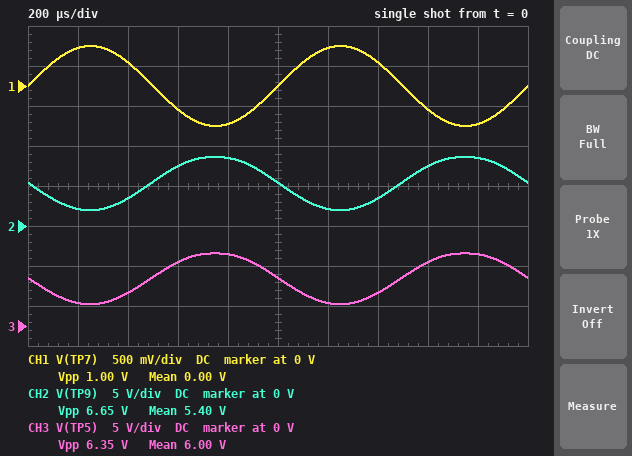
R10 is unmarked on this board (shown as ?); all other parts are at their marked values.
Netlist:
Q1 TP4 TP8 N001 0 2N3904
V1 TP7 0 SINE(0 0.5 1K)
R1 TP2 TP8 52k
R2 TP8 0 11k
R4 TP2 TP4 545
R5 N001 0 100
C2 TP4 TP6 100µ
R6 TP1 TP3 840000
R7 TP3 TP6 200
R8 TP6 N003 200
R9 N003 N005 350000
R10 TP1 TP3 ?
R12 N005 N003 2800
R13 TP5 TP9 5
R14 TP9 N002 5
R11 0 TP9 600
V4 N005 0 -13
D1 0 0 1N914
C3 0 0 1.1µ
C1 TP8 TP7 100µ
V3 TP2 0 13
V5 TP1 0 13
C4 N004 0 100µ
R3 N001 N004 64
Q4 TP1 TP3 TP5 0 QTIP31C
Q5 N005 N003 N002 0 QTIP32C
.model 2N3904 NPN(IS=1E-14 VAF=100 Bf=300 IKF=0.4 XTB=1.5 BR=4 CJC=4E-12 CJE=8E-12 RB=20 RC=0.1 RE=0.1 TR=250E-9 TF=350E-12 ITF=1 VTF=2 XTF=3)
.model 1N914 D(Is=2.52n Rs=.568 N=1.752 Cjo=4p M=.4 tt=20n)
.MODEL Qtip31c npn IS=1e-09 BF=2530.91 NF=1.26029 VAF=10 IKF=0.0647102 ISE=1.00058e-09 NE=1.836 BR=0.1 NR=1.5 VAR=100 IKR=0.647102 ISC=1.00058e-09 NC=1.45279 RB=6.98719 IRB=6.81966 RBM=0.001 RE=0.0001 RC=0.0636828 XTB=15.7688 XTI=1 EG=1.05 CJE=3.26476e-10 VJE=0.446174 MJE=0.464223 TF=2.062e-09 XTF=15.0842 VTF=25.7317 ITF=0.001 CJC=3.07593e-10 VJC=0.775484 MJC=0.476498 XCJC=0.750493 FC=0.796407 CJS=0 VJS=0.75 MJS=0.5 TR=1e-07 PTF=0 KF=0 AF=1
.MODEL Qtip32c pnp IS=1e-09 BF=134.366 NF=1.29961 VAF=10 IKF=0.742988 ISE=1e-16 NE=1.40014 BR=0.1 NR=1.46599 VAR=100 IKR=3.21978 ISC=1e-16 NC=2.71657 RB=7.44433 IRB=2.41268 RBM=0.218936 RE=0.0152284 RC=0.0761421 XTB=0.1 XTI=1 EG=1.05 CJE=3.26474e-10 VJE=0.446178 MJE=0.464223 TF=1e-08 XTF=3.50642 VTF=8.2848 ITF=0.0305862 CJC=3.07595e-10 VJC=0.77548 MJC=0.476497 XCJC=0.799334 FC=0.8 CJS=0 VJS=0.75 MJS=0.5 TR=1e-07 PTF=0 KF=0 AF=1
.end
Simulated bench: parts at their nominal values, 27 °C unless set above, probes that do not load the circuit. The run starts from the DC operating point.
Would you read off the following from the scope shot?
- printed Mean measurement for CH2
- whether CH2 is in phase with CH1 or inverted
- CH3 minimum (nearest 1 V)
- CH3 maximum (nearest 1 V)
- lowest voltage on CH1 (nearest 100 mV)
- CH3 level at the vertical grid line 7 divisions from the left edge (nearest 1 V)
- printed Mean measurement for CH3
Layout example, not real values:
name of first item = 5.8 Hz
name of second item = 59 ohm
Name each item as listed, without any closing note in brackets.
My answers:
printed Mean measurement for CH2 = 5.40 V
whether CH2 is in phase with CH1 or inverted = inverted
CH3 minimum = 3 V
CH3 maximum = 9 V
lowest voltage on CH1 = -500 mV
CH3 level at the vertical grid line 7 divisions from the left edge = 4 V
printed Mean measurement for CH3 = 6.00 V
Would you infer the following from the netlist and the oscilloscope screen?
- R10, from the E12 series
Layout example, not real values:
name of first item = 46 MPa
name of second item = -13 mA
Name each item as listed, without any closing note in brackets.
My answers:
R10, from the E12 series = 1 kΩ
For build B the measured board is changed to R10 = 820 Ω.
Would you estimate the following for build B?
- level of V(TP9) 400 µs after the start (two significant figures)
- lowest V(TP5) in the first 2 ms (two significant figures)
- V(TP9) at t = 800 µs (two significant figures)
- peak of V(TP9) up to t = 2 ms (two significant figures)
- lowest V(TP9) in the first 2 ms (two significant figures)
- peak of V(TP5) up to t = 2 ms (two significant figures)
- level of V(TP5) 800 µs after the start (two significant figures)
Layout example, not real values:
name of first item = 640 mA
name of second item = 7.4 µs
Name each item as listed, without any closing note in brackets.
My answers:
level of V(TP9) 400 µs after the start = 4.4 V
lowest V(TP5) in the first 2 ms = 3.8 V
V(TP9) at t = 800 µs = 9.1 V
peak of V(TP9) up to t = 2 ms = 9.2 V
lowest V(TP9) in the first 2 ms = 3.0 V
peak of V(TP5) up to t = 2 ms = 9.7 V
level of V(TP5) 800 µs after the start = 9.6 V
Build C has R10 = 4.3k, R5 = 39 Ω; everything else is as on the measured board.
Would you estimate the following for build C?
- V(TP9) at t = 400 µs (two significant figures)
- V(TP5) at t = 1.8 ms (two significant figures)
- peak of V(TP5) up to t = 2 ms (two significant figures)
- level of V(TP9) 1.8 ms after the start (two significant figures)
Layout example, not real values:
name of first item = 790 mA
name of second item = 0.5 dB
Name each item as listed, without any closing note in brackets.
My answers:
V(TP9) at t = 400 µs = -2.8 V
V(TP5) at t = 1.8 ms = 5.1 V
peak of V(TP5) up to t = 2 ms = 5.4 V
level of V(TP9) 1.8 ms after the start = 4.9 V
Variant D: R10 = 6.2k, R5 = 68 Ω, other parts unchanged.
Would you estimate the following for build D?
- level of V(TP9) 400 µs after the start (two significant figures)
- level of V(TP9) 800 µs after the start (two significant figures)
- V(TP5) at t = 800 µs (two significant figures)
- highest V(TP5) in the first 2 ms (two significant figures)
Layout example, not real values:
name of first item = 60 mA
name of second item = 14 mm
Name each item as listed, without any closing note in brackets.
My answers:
level of V(TP9) 400 µs after the start = -7.5 V
level of V(TP9) 800 µs after the start = 700 mV
V(TP5) at t = 800 µs = 810 mV
highest V(TP5) in the first 2 ms = 1.1 V
